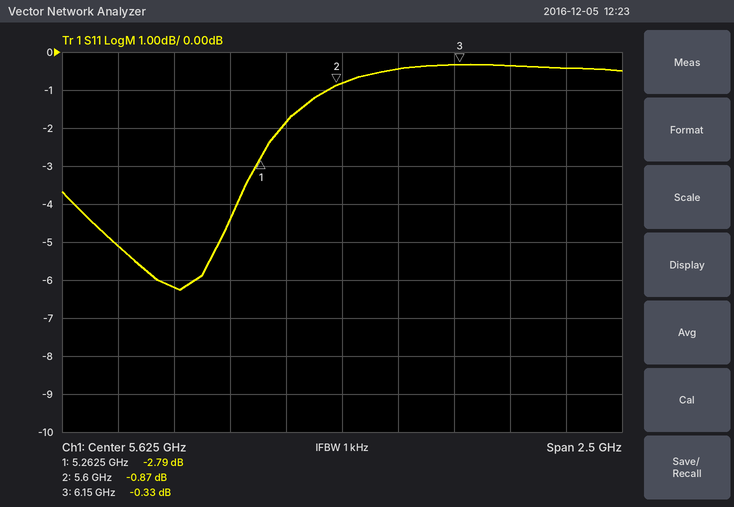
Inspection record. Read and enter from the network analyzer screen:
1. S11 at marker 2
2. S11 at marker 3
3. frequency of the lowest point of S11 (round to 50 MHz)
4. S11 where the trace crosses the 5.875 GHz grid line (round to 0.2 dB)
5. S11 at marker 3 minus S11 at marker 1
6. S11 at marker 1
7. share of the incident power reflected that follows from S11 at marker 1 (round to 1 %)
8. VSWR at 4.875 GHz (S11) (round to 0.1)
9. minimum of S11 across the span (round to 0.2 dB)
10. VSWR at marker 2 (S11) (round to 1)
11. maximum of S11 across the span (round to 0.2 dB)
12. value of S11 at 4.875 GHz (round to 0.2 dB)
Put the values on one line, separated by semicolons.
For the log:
-0.87 dB; -0.33 dB; 4.90 GHz; -0.4 dB; 2.46 dB; -2.79 dB; 53 %; 2.9; -6.2 dB; 20; -0.4 dB; -6.2 dB
